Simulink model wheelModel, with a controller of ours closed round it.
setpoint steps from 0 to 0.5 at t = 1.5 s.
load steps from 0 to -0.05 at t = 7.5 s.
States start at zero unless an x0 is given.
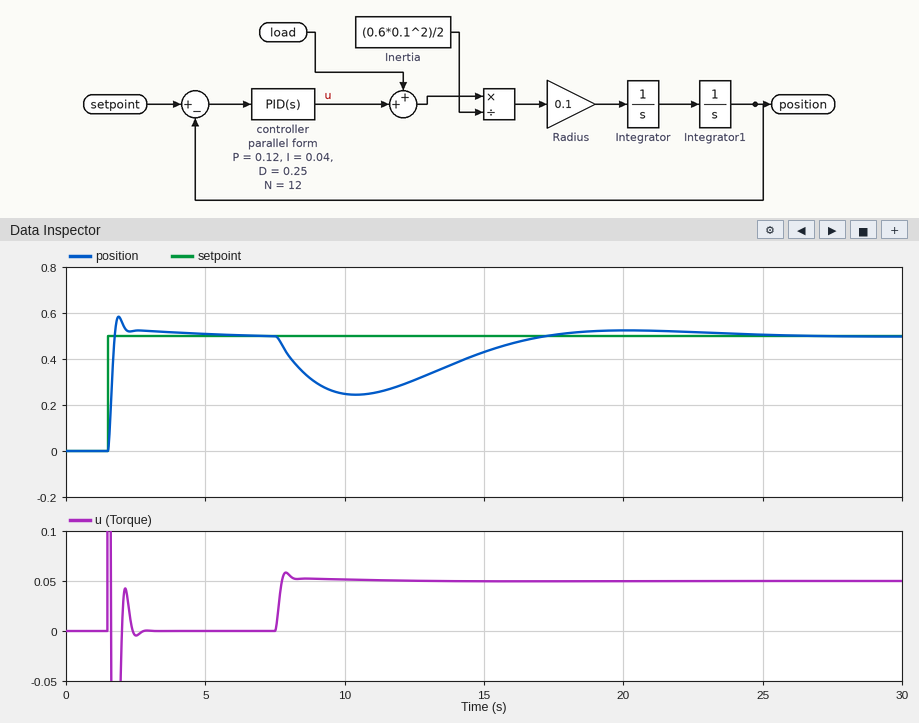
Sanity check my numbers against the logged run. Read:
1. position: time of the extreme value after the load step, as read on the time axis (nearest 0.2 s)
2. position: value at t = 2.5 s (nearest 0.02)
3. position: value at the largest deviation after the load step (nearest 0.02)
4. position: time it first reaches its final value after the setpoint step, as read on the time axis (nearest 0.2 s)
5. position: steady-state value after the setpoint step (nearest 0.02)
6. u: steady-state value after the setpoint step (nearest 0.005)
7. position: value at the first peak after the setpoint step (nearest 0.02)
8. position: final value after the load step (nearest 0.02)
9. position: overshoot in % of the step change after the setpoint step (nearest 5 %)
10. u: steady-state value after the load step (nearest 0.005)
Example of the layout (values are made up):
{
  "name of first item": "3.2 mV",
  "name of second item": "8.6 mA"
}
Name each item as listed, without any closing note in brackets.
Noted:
{
  "position: time of the extreme value after the load step, as read on the time axis": "10.4 s",
  "position: value at t = 2.5 s": "0.52",
  "position: value at the largest deviation after the load step": "0.24",
  "position: time it first reaches its final value after the setpoint step, as read on the time axis": "1.8 s",
  "position: steady-state value after the setpoint step": "0.50",
  "u: steady-state value after the setpoint step": "0.000",
  "position: value at the first peak after the setpoint step": "0.58",
  "position: final value after the load step": "0.50",
  "position: overshoot in % of the step change after the setpoint step": "15 %",
  "u: steady-state value after the load step": "0.050"
}
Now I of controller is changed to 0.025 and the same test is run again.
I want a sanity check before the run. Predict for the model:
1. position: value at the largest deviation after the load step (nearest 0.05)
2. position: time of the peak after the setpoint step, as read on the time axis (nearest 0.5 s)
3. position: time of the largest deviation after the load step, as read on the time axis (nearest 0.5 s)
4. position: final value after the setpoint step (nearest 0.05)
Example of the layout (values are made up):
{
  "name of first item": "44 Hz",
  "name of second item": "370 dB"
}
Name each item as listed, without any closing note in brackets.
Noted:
{
  "position: value at the largest deviation after the load step": "0.20",
  "position: time of the peak after the setpoint step, as read on the time axis": "2.0 s",
  "position: time of the largest deviation after the load step, as read on the time axis": "11.0 s",
  "position: final value after the setpoint step": "0.50"
}
